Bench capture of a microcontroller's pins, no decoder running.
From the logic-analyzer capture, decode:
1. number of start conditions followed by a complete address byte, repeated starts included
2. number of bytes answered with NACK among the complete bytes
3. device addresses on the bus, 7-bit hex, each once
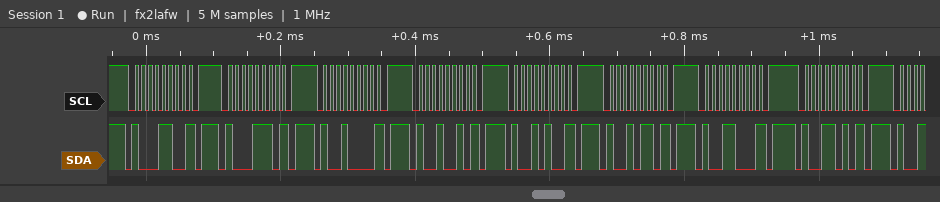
8
8
0x46 0x47 0x48 0x49 0x4A 0x4B 0x4C 0x4D
